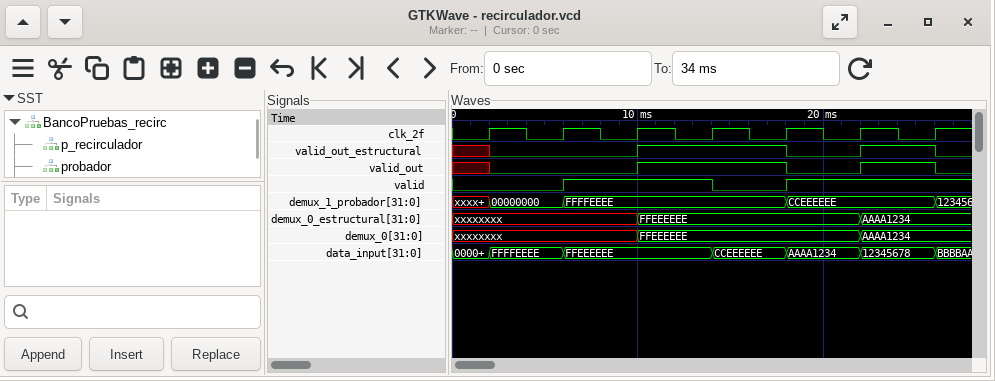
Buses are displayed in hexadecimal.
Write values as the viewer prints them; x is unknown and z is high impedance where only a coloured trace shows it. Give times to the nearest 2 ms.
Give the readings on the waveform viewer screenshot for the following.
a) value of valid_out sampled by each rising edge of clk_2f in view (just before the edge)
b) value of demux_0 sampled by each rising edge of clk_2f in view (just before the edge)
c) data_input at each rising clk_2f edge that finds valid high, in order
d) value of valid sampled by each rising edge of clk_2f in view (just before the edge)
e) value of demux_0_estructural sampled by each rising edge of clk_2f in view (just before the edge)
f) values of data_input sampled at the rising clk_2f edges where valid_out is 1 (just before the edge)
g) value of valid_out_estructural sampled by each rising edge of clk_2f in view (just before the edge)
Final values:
x 0 0 1 1 0 1
xxxxxxxx, xxxxxxxx, xxxxxxxx, FFEEEEEE, FFEEEEEE, FFEEEEEE, AAAA1234
FFEEEEEE, FFEEEEEE, AAAA1234, 12345678
0 0 1 1 0 1 1
xxxxxxxx, xxxxxxxx, xxxxxxxx, FFEEEEEE, FFEEEEEE, FFEEEEEE, AAAA1234
FFEEEEEE, CCEEEEEE, 12345678
x 0 0 1 1 0 1
